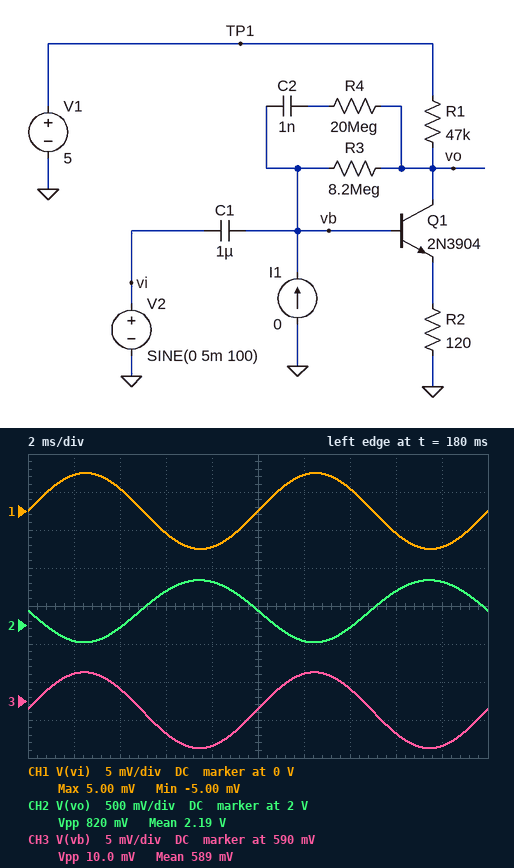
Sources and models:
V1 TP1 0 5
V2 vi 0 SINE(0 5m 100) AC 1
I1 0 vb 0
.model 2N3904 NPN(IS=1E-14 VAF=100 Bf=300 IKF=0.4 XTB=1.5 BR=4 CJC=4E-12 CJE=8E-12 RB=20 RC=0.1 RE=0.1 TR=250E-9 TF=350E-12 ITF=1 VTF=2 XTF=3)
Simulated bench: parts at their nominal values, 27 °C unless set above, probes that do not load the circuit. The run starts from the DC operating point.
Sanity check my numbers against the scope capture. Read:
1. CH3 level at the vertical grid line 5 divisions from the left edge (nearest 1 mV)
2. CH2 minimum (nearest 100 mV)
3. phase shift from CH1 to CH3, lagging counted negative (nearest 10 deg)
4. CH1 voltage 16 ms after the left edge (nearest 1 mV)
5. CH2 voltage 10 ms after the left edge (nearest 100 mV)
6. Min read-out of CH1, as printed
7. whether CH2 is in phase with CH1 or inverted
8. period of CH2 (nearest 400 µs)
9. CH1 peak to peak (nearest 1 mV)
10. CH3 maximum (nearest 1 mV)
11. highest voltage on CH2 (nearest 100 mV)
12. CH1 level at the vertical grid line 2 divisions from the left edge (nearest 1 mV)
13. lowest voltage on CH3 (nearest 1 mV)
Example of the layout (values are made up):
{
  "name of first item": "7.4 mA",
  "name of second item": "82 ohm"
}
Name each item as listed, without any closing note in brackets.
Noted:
{
  "CH3 level at the vertical grid line 5 divisions from the left edge": "589 mV",
  "CH2 minimum": "1.8 V",
  "phase shift from CH1 to CH3, lagging counted negative": "0 deg",
  "CH1 voltage 16 ms after the left edge": "-3 mV",
  "CH2 voltage 10 ms after the left edge": "2.2 V",
  "Min read-out of CH1, as printed": "-5.00 mV",
  "whether CH2 is in phase with CH1 or inverted": "inverted",
  "period of CH2": "10.0 ms",
  "CH1 peak to peak": "10 mV",
  "CH3 maximum": "594 mV",
  "highest voltage on CH2": "2.6 V",
  "CH1 level at the vertical grid line 2 divisions from the left edge": "3 mV",
  "lowest voltage on CH3": "584 mV"
}
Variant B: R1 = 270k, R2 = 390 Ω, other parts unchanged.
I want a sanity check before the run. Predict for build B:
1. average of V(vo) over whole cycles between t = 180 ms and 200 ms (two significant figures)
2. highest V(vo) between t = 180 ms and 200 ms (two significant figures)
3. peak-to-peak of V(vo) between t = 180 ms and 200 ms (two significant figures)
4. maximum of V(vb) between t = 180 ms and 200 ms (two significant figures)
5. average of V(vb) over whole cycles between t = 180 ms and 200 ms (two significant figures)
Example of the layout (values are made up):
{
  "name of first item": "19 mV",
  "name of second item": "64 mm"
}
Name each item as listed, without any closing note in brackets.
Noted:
{
  "average of V(vo) over whole cycles between t = 180 ms and 200 ms": "960 mV",
  "highest V(vo) between t = 180 ms and 200 ms": "1.5 V",
  "peak-to-peak of V(vo) between t = 180 ms and 200 ms": "1.2 V",
  "maximum of V(vb) between t = 180 ms and 200 ms": "560 mV",
  "average of V(vb) over whole cycles between t = 180 ms and 200 ms": "550 mV"
}
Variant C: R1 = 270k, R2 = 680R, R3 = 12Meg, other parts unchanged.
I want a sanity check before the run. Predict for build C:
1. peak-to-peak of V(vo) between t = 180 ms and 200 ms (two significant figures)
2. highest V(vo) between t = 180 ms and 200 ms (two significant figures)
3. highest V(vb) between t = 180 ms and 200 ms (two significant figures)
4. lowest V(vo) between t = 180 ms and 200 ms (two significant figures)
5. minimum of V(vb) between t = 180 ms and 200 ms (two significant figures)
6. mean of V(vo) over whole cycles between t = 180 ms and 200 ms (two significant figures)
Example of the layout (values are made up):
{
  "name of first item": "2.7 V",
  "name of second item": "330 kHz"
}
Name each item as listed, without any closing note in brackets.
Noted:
{
  "peak-to-peak of V(vo) between t = 180 ms and 200 ms": "1.0 V",
  "highest V(vo) between t = 180 ms and 200 ms": "1.6 V",
  "highest V(vb) between t = 180 ms and 200 ms": "560 mV",
  "lowest V(vo) between t = 180 ms and 200 ms": "600 mV",
  "minimum of V(vb) between t = 180 ms and 200 ms": "550 mV",
  "mean of V(vo) over whole cycles between t = 180 ms and 200 ms": "1.1 V"
}
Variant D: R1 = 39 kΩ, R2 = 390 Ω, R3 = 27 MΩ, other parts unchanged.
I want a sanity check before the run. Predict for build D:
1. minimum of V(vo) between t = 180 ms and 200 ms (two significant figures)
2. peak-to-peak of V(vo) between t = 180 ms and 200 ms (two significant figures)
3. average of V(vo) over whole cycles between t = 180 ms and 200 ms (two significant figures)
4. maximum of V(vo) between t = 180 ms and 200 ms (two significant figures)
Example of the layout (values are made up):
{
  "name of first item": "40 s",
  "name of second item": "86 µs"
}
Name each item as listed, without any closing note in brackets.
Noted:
{
  "minimum of V(vo) between t = 180 ms and 200 ms": "3.5 V",
  "peak-to-peak of V(vo) between t = 180 ms and 200 ms": "340 mV",
  "average of V(vo) over whole cycles between t = 180 ms and 200 ms": "3.6 V",
  "maximum of V(vo) between t = 180 ms and 200 ms": "3.8 V"
}
